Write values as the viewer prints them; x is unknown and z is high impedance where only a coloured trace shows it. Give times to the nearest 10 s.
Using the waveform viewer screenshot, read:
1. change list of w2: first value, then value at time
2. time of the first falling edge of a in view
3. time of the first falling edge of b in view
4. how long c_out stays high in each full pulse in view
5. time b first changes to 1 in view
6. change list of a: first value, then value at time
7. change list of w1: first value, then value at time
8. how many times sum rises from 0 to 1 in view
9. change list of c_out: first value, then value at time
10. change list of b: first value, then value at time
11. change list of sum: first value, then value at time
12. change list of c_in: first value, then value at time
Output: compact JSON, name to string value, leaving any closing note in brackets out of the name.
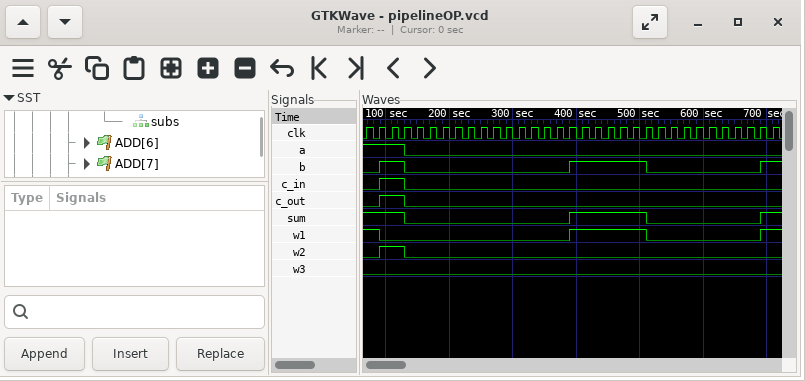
{"change list of w2: first value, then value at time": "0, 1 at 90 s, 0 at 130 s", "time of the first falling edge of a in view": "130 s", "time of the first falling edge of b in view": "130 s", "how long c_out stays high in each full pulse in view": "40 s", "time b first changes to 1 in view": "90 s", "change list of a: first value, then value at time": "1, 0 at 130 s", "change list of w1: first value, then value at time": "1, 0 at 90 s, 1 at 390 s, 0 at 510 s, 1 at 690 s", "how many times sum rises from 0 to 1 in view": "2", "change list of c_out: first value, then value at time": "0, 1 at 90 s, 0 at 130 s", "change list of b: first value, then value at time": "0, 1 at 90 s, 0 at 130 s, 1 at 390 s, 0 at 510 s, 1 at 690 s", "change list of sum: first value, then value at time": "1, 0 at 130 s, 1 at 390 s, 0 at 510 s, 1 at 690 s", "change list of c_in: first value, then value at time": "0, 1 at 90 s, 0 at 130 s"}
